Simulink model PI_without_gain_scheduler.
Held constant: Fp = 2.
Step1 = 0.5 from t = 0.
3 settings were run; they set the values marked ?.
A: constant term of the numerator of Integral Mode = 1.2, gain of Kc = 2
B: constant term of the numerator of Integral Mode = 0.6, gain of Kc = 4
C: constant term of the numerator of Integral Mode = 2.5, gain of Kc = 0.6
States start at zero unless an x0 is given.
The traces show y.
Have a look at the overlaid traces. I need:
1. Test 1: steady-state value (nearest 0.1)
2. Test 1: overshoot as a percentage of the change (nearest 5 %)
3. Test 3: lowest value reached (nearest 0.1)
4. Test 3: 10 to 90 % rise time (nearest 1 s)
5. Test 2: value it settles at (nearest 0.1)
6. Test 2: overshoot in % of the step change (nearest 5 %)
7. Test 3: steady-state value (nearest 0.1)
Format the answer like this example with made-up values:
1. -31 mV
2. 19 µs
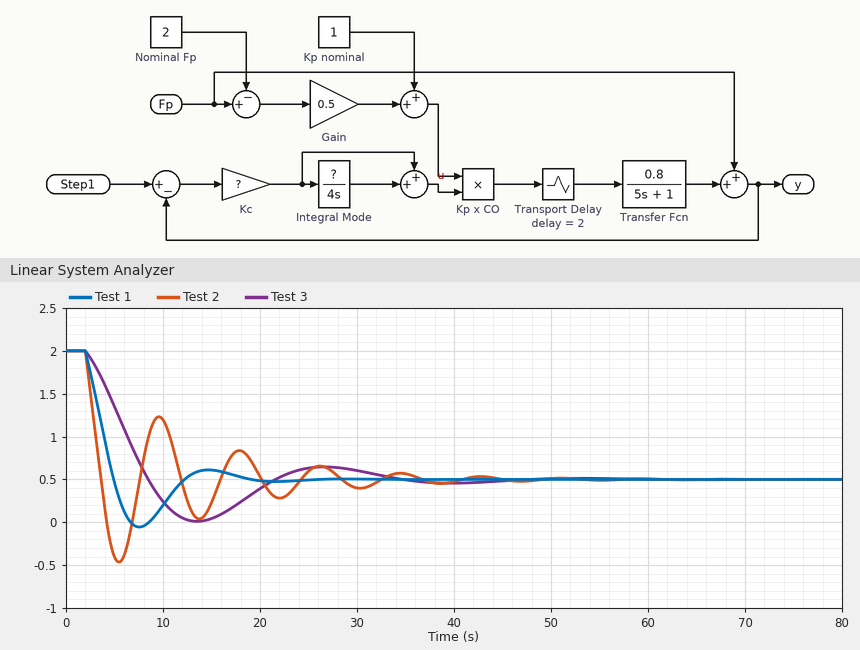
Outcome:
1. 0.5
2. 35 %
3. 0.0
4. 5 s
5. 0.5
6. 65 %
7. 0.5
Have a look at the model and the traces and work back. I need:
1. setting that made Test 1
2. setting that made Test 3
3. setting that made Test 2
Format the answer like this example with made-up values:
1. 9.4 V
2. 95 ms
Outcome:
1. A
2. C
3. B
